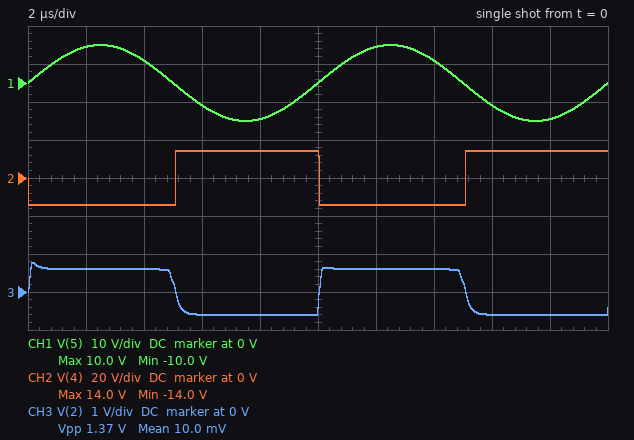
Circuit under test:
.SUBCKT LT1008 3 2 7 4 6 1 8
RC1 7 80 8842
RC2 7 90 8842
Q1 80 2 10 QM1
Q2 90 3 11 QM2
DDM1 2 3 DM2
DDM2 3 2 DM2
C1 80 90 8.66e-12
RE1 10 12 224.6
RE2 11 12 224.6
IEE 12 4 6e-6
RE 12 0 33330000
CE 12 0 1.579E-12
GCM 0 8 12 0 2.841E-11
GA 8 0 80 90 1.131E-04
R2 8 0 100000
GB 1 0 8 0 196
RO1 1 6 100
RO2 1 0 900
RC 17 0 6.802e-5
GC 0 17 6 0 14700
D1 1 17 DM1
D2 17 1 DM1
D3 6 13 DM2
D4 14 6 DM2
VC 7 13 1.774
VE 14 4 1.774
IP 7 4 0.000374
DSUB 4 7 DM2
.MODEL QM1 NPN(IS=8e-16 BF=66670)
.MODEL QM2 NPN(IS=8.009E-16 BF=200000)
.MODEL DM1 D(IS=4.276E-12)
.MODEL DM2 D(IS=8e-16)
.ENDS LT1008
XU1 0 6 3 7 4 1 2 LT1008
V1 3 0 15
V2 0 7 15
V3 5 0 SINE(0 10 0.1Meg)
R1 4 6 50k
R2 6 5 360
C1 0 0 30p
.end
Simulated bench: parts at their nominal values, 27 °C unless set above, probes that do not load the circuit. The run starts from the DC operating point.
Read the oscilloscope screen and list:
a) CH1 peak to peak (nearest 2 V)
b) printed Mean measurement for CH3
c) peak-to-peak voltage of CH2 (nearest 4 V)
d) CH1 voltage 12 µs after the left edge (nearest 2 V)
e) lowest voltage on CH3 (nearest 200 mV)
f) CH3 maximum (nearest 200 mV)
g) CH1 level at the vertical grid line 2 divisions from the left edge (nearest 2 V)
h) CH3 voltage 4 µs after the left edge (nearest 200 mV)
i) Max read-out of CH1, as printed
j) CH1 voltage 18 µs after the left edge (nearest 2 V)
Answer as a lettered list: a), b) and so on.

a) 20 V
b) 10.0 mV
c) 28 V
d) 10 V
e) -600 mV
f) 800 mV
g) 6 V
h) 600 mV
i) 10.0 V
j) -10 V
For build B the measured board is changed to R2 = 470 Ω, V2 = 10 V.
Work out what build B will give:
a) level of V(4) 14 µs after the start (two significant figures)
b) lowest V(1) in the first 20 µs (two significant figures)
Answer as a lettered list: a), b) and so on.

a) -9.0 V
b) -9.8 V
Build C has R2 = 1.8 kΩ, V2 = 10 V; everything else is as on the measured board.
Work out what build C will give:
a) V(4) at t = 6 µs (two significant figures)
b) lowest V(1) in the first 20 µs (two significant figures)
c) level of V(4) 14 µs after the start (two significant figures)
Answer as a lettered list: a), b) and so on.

a) 14 V
b) -9.8 V
c) -9.0 V
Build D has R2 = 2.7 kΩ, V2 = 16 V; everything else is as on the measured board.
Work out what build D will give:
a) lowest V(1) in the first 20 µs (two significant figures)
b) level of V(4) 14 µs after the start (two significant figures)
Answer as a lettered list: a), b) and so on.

a) -16 V
b) -15 V
